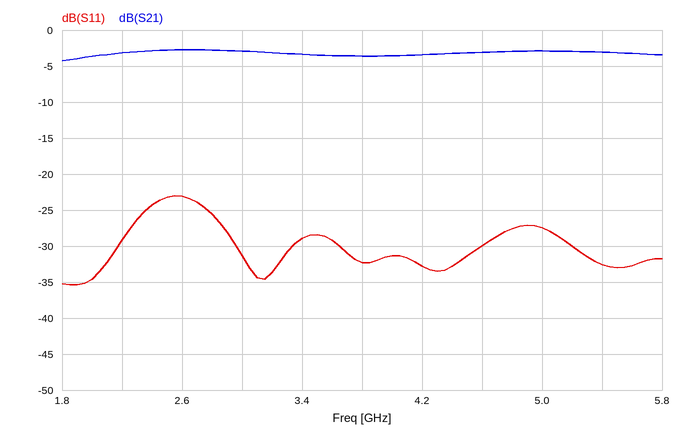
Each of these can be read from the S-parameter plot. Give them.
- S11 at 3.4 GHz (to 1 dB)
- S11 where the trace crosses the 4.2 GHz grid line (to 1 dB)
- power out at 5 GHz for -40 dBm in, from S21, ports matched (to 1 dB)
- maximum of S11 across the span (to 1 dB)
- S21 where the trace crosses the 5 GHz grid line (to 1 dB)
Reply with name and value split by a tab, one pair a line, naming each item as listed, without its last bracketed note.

S11 at 3.4 GHz	-29 dB
S11 where the trace crosses the 4.2 GHz grid line	-33 dB
power out at 5 GHz for -40 dBm in, from S21, ports matched	-43 dBm
maximum of S11 across the span	-23 dB
S21 where the trace crosses the 5 GHz grid line	-3 dB
